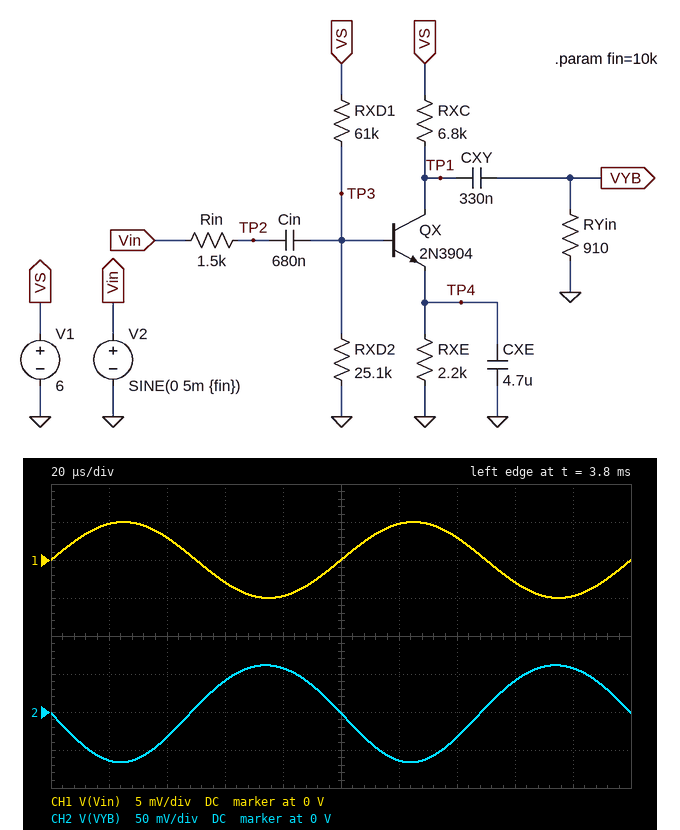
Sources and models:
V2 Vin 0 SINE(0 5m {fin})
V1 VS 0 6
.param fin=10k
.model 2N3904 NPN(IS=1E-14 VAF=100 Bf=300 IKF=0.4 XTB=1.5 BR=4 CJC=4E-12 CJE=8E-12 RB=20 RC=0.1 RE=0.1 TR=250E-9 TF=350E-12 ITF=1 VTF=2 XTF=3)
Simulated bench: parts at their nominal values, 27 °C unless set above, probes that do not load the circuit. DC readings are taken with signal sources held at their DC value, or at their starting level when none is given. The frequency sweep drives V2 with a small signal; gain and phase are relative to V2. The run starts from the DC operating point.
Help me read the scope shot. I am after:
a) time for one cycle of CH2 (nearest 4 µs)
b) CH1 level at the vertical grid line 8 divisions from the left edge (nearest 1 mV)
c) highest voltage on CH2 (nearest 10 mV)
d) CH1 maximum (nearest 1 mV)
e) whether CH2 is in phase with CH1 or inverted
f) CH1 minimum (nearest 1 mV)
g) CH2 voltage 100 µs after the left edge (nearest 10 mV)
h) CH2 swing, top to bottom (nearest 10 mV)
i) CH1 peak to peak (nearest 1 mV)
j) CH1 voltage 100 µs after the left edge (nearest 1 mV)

100 µs
-3 mV
60 mV
5 mV
inverted
-5 mV
0 V
130 mV
10 mV
0 V
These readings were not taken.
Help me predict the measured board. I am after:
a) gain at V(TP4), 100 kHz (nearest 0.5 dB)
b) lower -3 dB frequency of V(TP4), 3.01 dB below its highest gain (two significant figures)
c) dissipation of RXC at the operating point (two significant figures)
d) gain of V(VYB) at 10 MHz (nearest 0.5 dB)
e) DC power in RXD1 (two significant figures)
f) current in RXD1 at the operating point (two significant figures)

-45.5 dB
12 Hz
1.6 mW
7.0 dB
300 µW
70 µA
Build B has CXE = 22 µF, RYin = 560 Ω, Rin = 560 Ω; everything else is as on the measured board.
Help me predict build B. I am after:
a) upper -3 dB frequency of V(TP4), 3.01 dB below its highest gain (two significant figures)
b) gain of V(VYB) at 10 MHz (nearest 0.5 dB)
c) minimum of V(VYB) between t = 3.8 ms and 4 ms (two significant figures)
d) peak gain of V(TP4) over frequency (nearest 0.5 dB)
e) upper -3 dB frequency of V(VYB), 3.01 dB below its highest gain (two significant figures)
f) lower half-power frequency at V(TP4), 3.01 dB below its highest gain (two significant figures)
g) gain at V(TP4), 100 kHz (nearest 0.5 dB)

170 Hz
13.0 dB
-47 mV
-2.0 dB
5.4 MHz
10 Hz
-58.0 dB
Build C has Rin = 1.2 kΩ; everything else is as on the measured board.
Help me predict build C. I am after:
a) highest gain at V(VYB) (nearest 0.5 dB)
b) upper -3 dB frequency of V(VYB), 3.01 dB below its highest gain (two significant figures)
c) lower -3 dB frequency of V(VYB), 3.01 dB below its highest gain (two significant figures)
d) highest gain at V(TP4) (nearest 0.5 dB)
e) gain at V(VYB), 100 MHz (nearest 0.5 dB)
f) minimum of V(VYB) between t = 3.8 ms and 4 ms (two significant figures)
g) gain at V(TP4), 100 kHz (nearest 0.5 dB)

22.5 dB
2.1 MHz
630 Hz
-1.0 dB
-11.5 dB
-68 mV
-45.0 dB
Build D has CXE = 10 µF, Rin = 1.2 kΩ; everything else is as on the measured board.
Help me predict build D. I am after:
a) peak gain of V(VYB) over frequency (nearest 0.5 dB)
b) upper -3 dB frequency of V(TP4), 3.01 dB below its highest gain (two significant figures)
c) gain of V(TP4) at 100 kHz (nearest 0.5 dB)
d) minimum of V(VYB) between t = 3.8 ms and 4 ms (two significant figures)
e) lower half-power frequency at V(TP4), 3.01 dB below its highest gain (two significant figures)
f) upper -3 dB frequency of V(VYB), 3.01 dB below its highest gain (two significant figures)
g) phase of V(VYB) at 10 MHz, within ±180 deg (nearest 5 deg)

22.5 dB
320 Hz
-51.5 dB
-68 mV
11 Hz
2.1 MHz
100 deg
